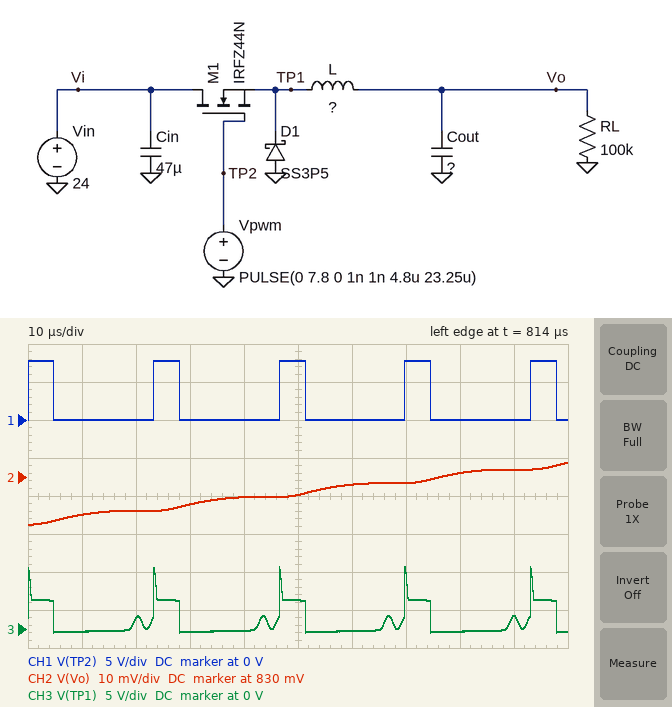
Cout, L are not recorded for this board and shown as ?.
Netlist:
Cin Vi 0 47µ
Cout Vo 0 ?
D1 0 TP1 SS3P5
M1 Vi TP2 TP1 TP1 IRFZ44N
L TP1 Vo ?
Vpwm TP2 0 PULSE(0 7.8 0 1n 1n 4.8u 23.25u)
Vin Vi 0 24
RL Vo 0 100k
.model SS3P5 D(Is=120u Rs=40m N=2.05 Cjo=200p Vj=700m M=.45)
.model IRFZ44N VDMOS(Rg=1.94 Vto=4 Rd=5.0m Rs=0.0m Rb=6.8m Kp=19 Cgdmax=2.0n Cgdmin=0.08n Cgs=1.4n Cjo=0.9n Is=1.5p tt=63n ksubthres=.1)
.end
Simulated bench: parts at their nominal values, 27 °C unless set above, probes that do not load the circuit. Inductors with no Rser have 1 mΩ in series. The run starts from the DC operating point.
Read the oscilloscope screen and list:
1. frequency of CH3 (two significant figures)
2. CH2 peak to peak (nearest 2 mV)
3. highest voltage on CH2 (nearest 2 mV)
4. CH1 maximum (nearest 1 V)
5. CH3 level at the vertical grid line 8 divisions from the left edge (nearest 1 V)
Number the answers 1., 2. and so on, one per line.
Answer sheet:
1. 43 kHz
2. 16 mV
3. 834 mV
4. 8 V
5. 0 V
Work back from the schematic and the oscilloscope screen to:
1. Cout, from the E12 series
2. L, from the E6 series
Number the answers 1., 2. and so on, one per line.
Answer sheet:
1. 270 µF
2. 150 µH
